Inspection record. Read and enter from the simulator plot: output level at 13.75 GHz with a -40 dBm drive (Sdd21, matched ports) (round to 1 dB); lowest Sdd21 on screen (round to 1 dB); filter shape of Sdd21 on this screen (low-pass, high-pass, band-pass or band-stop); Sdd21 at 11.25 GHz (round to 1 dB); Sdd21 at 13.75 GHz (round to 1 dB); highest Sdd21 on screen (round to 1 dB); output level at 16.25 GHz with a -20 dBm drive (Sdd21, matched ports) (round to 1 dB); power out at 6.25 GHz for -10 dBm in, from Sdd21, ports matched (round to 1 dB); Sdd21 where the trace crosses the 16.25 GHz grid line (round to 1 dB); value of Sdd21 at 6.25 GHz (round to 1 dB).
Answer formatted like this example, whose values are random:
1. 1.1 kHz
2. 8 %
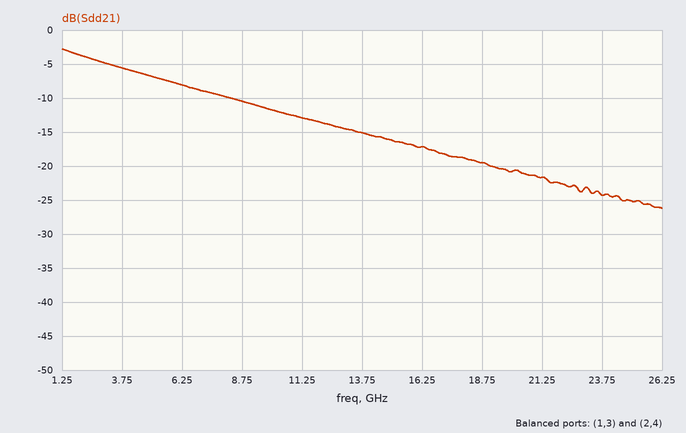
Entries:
1. -55 dBm
2. -26 dB
3. low-pass
4. -13 dB
5. -15 dB
6. -3 dB
7. -37 dBm
8. -18 dBm
9. -17 dB
10. -8 dB
